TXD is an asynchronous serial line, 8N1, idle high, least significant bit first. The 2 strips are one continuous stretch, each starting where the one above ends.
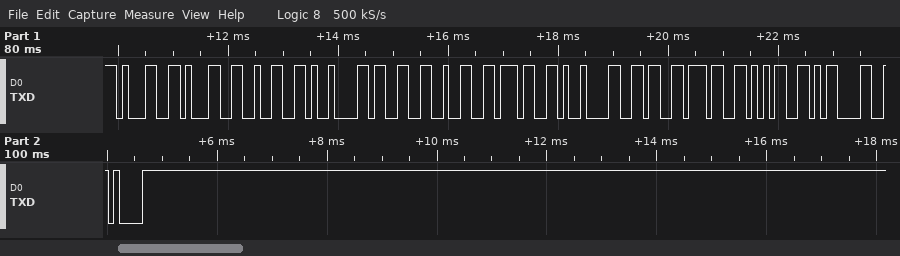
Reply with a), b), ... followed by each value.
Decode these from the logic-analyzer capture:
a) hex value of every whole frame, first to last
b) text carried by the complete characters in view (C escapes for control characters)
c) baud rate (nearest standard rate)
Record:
a) 31 31 32 09 33 32 37 09 36 37 35 0D 0A
b) "112\t327\t675\r\n"
c) 9600 baud
